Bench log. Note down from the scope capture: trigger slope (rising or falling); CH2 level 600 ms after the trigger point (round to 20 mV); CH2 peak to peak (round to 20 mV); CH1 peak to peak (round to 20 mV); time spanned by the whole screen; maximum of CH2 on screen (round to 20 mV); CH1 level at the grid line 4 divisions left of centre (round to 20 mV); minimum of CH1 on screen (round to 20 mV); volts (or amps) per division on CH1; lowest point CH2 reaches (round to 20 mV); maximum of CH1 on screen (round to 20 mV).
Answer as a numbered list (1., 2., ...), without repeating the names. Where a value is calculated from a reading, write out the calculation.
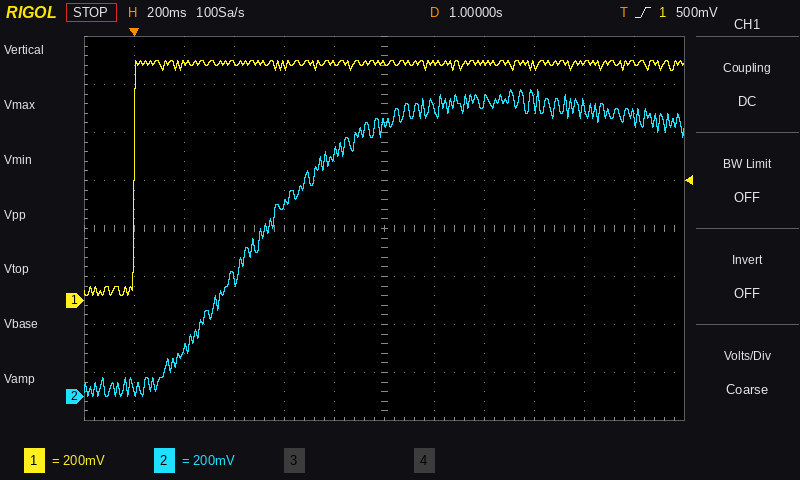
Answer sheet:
1. rising
2. 800 mV
3. 1.28 V − (0 mV) = 1.28 V
4. 1.00 V − (20 mV) = 980 mV
5. 2.4 s
6. 1.28 V
7. 980 mV
8. 20 mV
9. 200 mV
10. 0 mV
11. 1.00 V
